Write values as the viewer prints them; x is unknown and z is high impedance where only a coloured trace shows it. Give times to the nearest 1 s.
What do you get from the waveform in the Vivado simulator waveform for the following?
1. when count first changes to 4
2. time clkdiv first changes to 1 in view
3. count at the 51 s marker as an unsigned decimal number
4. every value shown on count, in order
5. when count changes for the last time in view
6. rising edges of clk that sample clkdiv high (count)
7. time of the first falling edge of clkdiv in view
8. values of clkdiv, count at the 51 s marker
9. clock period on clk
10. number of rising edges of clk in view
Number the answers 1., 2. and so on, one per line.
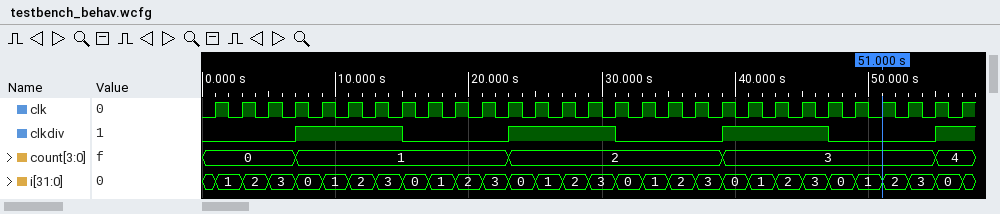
1. 55 s
2. 7 s
3. 3
4. 0, 1, 2, 3, 4
5. 55 s
6. 13
7. 15 s
8. clkdiv=0, count=3
9. 2 s
10. 29
